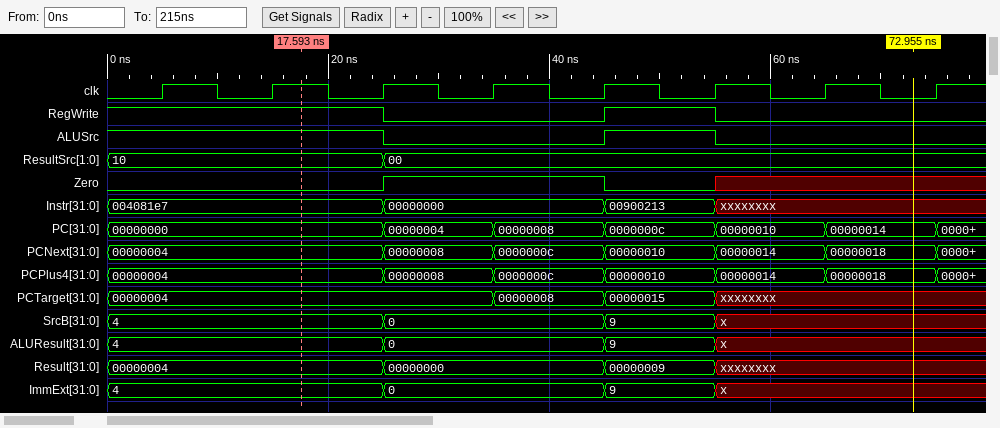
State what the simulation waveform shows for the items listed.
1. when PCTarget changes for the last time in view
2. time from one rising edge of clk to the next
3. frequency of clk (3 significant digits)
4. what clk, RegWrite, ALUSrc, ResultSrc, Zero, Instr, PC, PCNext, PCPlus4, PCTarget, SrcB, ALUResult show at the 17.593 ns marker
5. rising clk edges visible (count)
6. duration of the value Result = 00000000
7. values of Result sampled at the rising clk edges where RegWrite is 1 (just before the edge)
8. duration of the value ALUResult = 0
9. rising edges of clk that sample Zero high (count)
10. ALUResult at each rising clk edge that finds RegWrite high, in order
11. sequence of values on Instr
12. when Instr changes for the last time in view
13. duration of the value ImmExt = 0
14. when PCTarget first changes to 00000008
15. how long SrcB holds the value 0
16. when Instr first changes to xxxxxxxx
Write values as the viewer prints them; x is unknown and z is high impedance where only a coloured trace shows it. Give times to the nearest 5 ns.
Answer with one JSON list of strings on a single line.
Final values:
["55 ns", "10 ns", "100 MHz", "clk=1, RegWrite=1, ALUSrc=1, ResultSrc=10, Zero=0, Instr=004081e7, PC=00000000, PCNext=00000004, PCPlus4=00000004, PCTarget=00000004, SrcB=4, ALUResult=4", "8", "20 ns", "00000004, 00000004, 00000004, 00000009", "20 ns", "2", "4, 4, 4, 9", "004081e7, 00000000, 00900213, xxxxxxxx", "55 ns", "20 ns", "35 ns", "20 ns", "55 ns"]
